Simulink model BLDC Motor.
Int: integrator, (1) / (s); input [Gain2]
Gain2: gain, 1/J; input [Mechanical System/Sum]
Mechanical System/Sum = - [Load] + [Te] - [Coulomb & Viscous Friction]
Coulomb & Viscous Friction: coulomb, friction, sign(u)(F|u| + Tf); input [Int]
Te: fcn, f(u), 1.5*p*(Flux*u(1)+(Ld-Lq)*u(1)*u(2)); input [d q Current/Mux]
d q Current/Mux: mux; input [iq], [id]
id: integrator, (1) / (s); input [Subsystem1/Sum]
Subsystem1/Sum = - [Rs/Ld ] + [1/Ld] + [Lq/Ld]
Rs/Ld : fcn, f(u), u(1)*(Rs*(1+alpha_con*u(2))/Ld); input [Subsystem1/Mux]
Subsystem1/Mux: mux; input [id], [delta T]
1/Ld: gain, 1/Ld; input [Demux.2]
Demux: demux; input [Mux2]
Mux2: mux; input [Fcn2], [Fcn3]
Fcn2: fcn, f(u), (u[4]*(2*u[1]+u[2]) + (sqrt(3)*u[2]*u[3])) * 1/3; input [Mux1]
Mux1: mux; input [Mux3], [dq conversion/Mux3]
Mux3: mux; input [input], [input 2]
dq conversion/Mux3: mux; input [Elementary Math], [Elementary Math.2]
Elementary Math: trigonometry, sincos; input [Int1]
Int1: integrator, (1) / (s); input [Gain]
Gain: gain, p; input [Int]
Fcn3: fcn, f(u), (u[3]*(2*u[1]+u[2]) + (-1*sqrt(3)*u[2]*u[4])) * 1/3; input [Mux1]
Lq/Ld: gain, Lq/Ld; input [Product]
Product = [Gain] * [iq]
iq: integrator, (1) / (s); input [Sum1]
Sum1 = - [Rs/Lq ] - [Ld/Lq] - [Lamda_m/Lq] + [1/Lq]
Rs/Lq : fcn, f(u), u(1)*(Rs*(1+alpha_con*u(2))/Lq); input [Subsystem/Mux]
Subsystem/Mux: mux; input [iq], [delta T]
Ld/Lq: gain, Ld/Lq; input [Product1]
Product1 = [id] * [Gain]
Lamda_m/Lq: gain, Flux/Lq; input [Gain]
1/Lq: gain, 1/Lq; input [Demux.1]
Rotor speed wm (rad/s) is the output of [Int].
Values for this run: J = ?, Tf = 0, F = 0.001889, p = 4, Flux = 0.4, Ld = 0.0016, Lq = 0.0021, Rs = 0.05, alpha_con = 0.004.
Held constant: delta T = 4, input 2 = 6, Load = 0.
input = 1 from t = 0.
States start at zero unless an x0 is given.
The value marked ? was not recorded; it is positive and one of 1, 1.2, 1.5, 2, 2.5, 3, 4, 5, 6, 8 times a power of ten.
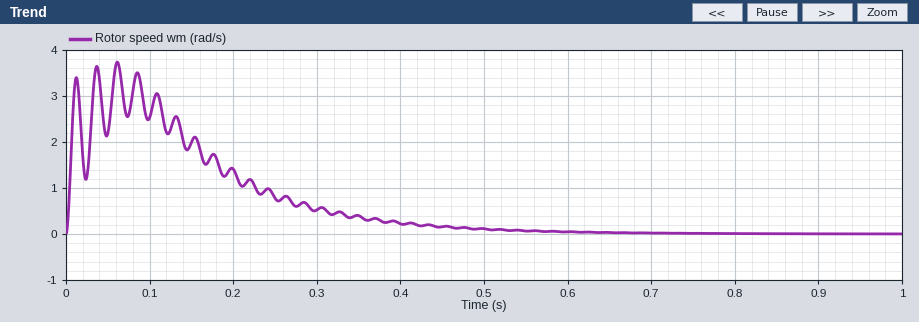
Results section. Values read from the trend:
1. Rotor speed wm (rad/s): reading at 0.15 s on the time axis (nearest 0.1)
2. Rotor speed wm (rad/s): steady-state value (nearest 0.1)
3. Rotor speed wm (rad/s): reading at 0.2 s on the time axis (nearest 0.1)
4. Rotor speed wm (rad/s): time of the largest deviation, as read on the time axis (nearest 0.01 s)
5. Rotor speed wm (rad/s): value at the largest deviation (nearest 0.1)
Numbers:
2.0
0.0
1.4
0.06 s
3.7
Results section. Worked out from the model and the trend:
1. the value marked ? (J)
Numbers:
0.025
